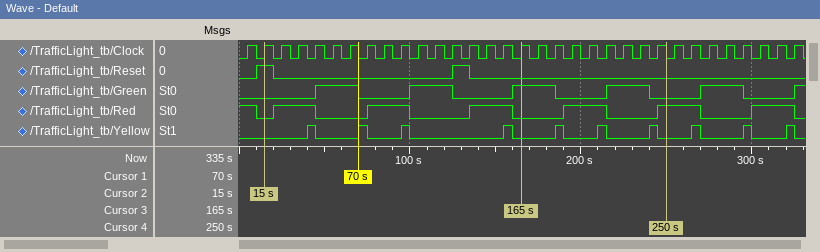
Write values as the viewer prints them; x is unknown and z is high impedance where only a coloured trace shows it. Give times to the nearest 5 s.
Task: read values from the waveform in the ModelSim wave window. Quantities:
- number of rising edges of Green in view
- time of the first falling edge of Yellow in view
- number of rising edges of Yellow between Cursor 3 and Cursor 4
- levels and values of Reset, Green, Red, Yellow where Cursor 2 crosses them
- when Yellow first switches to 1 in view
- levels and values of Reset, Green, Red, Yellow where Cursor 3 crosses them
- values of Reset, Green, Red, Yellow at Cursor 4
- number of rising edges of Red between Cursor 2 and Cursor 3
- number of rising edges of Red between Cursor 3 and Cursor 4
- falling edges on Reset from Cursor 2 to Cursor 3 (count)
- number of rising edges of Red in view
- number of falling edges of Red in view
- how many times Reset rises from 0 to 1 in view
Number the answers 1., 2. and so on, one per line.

1. 6
2. 45 s
3. 3
4. Reset=1, Green=0, Red=0, Yellow=0
5. 40 s
6. Reset=0, Green=1, Red=0, Yellow=0
7. Reset=0, Green=0, Red=1, Yellow=0
8. 3
9. 2
10. 2
11. 6
12. 7
13. 2
